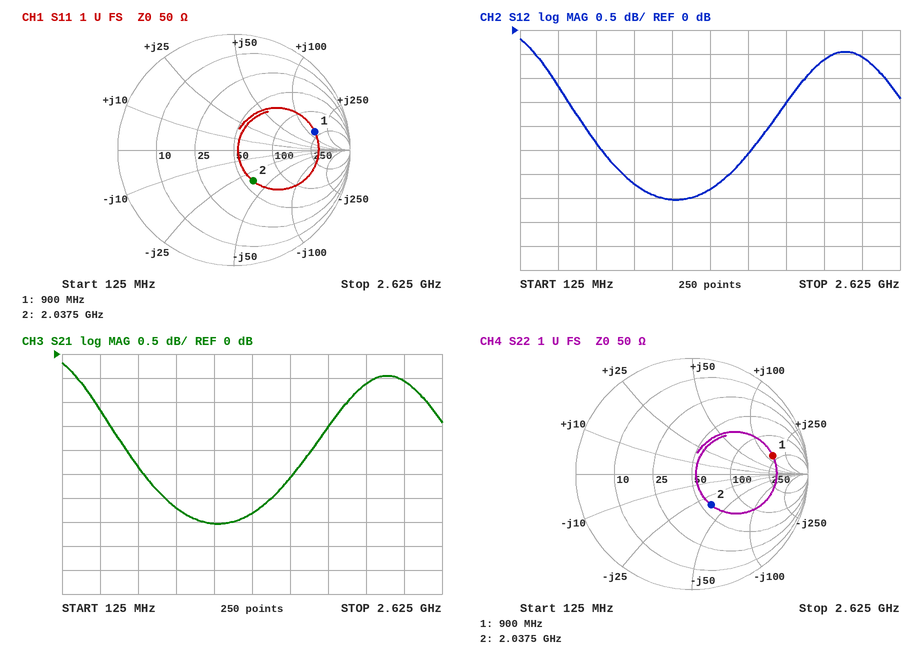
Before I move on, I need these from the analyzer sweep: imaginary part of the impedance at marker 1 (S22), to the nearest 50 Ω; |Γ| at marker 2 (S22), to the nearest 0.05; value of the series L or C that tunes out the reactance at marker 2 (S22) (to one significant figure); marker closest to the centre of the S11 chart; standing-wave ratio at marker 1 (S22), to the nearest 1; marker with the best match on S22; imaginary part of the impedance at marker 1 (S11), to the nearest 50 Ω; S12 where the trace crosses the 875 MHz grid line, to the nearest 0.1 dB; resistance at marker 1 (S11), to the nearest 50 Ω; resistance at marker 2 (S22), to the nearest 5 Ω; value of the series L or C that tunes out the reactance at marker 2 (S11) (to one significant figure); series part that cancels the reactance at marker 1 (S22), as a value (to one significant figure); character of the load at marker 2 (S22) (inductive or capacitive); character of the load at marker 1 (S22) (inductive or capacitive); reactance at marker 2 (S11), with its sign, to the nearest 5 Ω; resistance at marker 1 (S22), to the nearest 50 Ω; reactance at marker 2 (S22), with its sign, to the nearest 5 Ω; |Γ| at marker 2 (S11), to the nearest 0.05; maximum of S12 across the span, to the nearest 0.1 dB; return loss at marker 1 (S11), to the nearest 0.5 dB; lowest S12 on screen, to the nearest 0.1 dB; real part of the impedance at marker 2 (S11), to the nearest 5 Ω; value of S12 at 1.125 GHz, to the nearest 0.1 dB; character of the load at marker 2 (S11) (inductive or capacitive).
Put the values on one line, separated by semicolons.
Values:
+150 Ω; 0.30; 3 nH; marker 2; 6; marker 2; +150 Ω; -3.2 dB; 200 Ω; 60 Ω; 3 nH; 1 pF; capacitive; inductive; -35 Ω; 200 Ω; -35 Ω; 0.30; -0.2 dB; 3.0 dB; -3.5 dB; 60 Ω; -3.5 dB; capacitive
